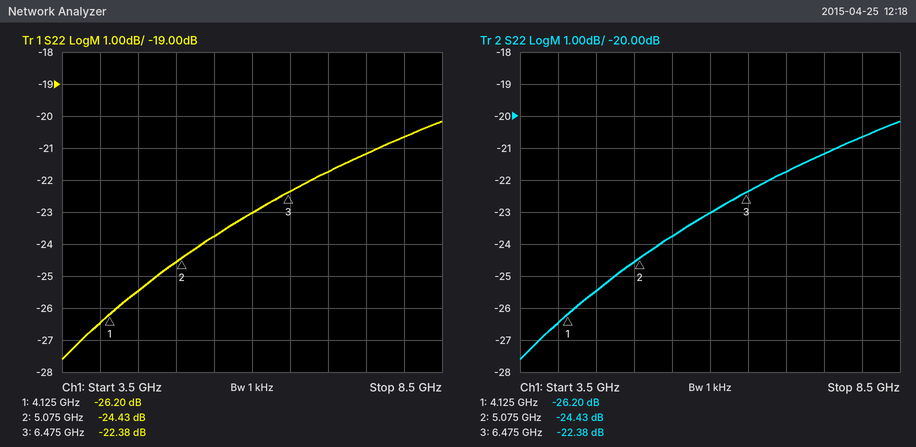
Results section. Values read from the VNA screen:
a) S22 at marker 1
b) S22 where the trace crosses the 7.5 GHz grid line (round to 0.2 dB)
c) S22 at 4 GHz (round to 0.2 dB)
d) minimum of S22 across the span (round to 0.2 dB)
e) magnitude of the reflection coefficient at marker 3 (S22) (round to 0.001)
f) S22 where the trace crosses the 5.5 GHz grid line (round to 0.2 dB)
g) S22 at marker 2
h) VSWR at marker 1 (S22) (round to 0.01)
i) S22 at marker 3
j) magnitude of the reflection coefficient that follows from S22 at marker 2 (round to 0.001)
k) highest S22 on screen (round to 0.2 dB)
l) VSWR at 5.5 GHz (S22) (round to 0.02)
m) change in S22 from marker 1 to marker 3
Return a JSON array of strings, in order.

["-26.20 dB", "-21.2 dB", "-26.4 dB", "-27.6 dB", "0.076", "-23.8 dB", "-24.43 dB", "1.10", "-22.38 dB", "0.060", "-20.2 dB", "1.14", "3.82 dB"]
